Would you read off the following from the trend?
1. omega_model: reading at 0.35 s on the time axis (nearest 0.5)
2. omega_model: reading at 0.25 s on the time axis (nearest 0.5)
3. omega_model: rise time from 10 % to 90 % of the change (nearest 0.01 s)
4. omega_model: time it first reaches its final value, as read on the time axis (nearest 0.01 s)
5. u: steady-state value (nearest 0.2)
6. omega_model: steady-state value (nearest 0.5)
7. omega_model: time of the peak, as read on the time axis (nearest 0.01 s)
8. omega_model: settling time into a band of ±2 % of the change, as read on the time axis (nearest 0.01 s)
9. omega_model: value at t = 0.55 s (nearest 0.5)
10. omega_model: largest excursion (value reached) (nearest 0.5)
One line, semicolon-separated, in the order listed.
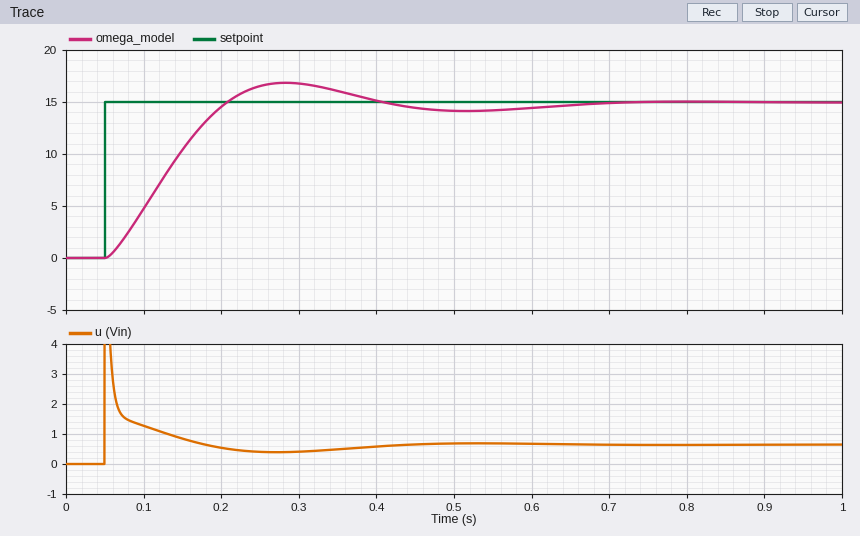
16.0; 16.5; 0.11 s; 0.21 s; 0.6; 15.0; 0.28 s; 0.65 s; 14.0; 17.0
